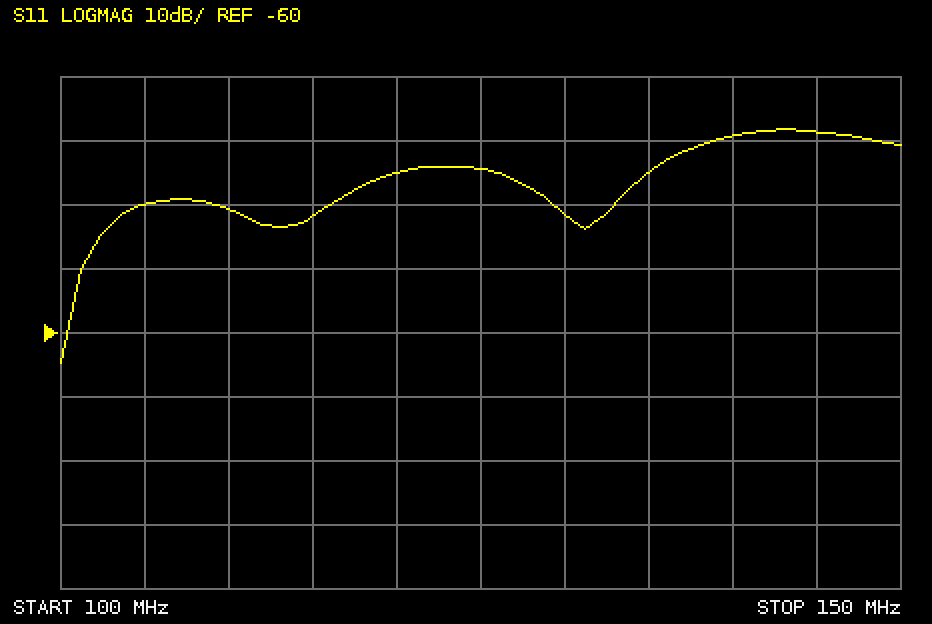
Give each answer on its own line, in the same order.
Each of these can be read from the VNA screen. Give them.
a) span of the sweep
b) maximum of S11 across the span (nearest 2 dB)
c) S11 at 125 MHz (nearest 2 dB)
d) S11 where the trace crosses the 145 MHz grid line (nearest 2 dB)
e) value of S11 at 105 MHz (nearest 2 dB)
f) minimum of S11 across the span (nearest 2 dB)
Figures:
50 MHz
-28 dB
-34 dB
-28 dB
-40 dB
-64 dB
